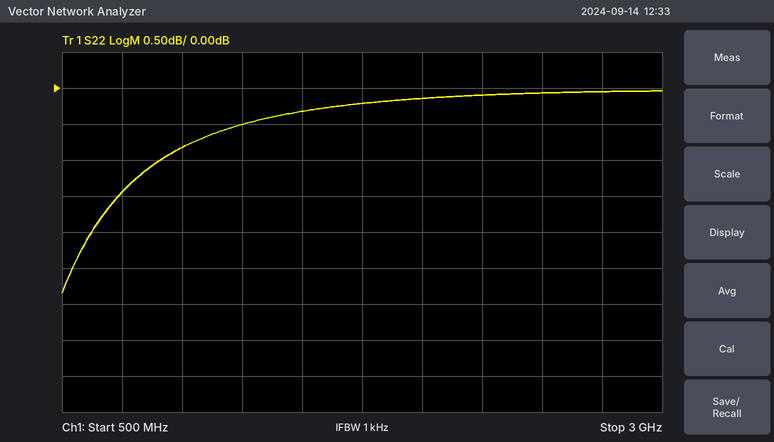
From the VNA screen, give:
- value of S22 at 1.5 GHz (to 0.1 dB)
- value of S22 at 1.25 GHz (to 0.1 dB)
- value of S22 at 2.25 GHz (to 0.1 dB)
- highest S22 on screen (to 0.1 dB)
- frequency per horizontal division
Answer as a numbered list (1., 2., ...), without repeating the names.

1. -0.3 dB
2. -0.5 dB
3. -0.1 dB
4. 0.0 dB
5. 250 MHz
